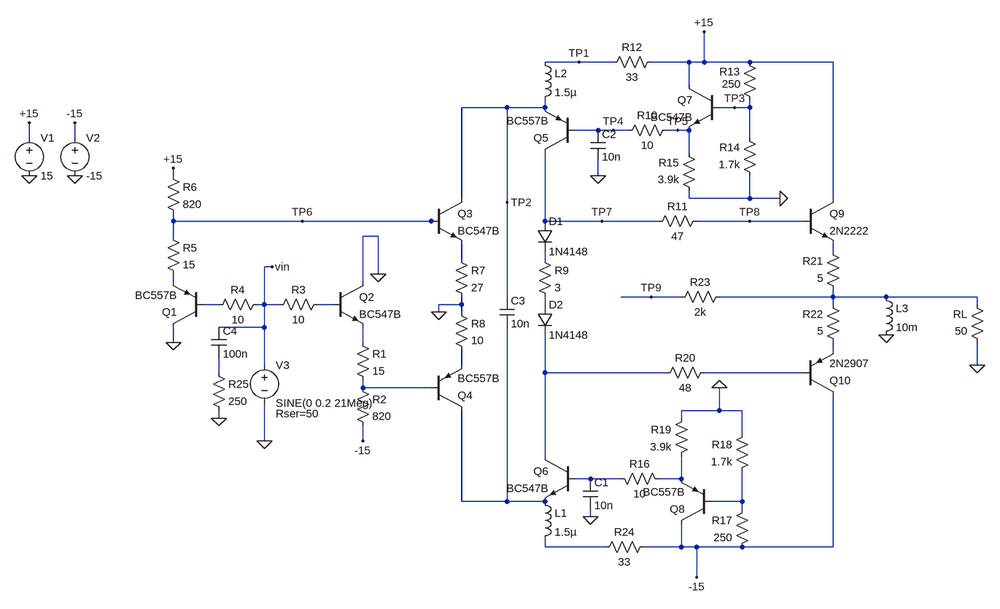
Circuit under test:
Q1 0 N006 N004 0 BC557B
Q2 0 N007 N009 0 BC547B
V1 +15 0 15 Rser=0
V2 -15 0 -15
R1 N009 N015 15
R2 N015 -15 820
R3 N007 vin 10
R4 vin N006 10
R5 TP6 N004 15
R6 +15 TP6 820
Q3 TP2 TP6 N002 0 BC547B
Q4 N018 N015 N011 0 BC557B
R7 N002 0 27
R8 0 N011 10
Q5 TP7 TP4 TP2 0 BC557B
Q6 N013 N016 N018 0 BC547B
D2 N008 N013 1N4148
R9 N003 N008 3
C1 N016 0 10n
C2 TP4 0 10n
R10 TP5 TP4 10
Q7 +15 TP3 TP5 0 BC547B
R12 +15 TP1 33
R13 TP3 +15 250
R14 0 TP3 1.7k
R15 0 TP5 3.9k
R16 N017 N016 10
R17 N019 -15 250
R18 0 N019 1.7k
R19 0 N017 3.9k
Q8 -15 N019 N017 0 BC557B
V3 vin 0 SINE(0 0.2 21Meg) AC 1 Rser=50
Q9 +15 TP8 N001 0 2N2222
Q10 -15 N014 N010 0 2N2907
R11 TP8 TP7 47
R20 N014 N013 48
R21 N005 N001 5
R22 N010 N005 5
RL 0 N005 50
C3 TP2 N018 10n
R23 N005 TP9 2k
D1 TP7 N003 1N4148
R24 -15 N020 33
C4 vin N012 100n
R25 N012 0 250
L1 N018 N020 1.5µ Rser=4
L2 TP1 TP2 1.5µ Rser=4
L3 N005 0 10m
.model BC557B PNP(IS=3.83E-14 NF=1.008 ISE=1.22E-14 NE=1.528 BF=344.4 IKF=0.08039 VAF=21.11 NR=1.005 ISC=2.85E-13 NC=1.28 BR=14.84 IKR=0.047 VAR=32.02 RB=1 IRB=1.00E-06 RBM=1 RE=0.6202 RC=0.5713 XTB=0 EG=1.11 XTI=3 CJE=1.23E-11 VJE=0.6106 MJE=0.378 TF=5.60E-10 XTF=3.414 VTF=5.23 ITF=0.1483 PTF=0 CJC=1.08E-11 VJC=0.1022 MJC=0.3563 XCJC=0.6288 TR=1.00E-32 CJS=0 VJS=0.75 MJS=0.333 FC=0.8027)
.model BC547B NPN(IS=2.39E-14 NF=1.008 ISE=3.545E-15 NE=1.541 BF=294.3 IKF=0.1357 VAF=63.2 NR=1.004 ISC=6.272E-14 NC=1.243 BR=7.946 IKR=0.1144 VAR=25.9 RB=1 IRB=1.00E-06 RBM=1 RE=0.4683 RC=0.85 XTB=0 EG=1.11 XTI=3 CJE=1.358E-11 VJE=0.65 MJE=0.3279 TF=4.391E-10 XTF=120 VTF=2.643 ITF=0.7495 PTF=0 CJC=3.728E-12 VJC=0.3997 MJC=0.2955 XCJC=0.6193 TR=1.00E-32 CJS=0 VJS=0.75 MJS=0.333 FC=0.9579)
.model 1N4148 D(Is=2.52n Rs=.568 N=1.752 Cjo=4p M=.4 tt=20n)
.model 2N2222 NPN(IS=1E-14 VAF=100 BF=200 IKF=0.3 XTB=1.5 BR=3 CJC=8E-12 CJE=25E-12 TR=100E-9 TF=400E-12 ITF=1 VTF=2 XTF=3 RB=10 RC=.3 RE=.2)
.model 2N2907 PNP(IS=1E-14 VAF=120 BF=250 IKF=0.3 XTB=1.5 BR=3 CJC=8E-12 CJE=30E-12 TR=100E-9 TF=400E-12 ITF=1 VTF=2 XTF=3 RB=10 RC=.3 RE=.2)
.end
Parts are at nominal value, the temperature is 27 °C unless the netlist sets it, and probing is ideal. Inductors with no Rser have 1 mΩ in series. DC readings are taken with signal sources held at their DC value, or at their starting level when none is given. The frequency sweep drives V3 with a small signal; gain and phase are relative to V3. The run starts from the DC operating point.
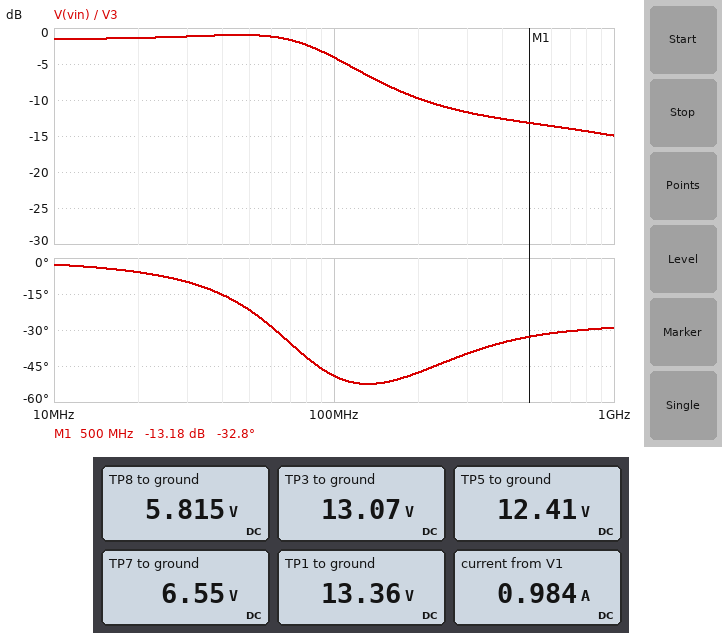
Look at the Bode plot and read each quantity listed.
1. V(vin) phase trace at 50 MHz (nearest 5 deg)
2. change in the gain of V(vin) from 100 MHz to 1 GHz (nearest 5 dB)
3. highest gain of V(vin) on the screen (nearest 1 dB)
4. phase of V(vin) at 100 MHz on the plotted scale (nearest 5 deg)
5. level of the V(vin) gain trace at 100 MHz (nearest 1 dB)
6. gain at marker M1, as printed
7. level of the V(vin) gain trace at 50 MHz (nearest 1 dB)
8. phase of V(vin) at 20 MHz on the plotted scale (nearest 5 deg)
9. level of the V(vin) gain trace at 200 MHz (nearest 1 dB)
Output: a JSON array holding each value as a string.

["-20 deg", "-10 dB", "-1 dB", "-50 deg", "-4 dB", "-13.18 dB", "-1 dB", "-5 deg", "-10 dB"]
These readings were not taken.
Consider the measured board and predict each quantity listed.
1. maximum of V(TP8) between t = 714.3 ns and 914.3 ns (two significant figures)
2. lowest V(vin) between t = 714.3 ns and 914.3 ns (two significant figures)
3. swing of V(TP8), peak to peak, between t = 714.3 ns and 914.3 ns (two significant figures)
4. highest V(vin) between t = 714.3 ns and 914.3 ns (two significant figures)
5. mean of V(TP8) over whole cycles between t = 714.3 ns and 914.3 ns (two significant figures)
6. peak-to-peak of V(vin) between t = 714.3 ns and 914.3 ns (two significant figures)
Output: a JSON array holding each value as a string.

["9.6 V", "-160 mV", "9.0 V", "170 mV", "5.7 V", "330 mV"]
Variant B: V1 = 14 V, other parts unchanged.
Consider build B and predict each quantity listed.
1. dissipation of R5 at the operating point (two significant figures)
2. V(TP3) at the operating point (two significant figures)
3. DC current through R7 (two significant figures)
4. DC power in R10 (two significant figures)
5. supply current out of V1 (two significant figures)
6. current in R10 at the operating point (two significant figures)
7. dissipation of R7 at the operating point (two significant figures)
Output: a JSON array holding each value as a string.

["3.8 mW", "12 V", "9.4 mA", "140 nW", "880 mA", "120 µA", "2.4 mW"]
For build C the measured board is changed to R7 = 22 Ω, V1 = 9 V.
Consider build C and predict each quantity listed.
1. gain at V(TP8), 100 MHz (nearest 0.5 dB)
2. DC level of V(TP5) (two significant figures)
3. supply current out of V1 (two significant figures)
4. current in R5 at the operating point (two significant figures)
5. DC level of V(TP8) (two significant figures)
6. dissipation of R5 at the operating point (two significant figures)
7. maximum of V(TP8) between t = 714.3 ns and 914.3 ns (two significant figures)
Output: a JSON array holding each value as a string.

["12.5 dB", "7.2 V", "46 mA", "9.9 mA", "-460 mV", "1.5 mW", "7.0 V"]
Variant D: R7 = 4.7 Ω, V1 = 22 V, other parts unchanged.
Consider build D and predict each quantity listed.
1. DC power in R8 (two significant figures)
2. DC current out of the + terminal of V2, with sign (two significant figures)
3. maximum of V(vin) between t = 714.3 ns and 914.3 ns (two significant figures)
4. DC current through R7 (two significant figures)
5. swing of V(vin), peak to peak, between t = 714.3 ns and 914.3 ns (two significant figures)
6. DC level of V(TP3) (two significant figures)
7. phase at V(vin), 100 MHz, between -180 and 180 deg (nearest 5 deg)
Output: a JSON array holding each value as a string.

["6.7 mW", "-1.1 A", "180 mV", "70 mA", "340 mV", "19 V", "-55 deg"]
